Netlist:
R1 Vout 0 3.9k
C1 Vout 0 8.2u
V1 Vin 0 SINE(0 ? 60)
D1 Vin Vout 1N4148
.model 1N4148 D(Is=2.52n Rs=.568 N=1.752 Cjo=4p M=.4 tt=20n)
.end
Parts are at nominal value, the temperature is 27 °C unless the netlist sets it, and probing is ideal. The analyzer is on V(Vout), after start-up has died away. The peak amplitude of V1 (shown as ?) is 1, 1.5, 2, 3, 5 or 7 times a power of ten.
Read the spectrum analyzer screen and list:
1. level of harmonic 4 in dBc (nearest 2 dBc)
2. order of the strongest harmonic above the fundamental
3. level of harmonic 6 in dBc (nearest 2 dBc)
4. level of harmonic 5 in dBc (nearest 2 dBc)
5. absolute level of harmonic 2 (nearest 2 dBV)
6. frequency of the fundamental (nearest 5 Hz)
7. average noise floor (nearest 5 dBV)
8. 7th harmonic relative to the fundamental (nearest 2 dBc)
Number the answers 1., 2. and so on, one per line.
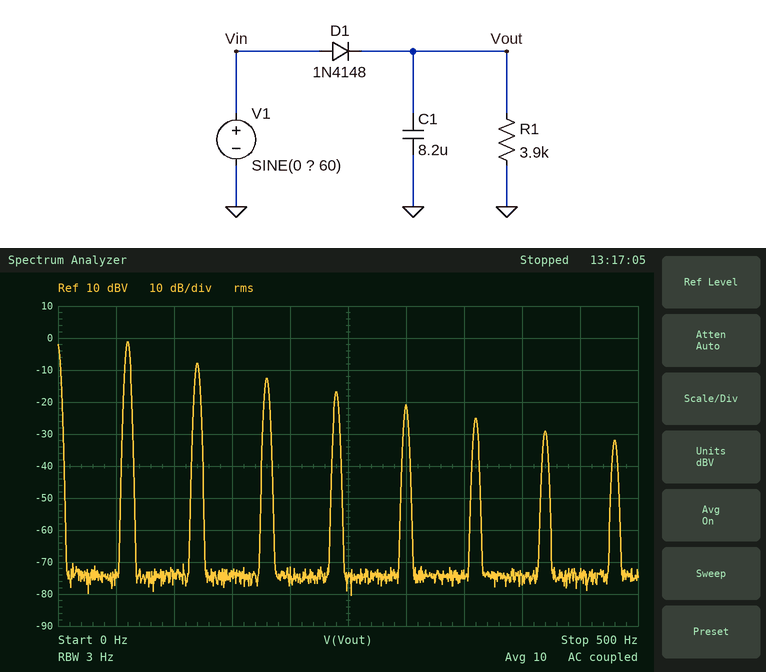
1. -16 dBc
2. 2
3. -24 dBc
4. -20 dBc
5. -8 dBV
6. 60 Hz
7. -75 dBV
8. -28 dBc
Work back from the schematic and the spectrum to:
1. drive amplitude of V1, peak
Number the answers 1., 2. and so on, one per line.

1. 10 V
